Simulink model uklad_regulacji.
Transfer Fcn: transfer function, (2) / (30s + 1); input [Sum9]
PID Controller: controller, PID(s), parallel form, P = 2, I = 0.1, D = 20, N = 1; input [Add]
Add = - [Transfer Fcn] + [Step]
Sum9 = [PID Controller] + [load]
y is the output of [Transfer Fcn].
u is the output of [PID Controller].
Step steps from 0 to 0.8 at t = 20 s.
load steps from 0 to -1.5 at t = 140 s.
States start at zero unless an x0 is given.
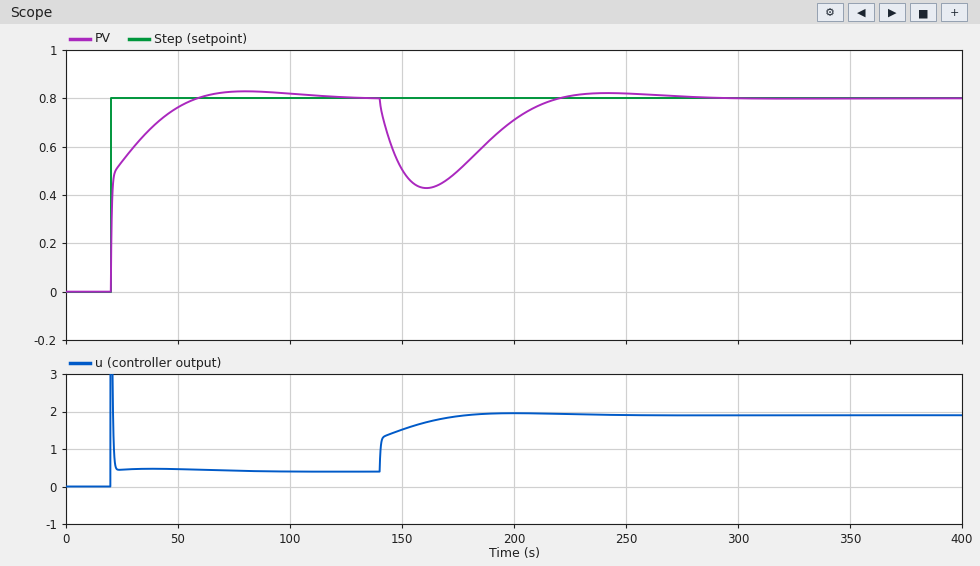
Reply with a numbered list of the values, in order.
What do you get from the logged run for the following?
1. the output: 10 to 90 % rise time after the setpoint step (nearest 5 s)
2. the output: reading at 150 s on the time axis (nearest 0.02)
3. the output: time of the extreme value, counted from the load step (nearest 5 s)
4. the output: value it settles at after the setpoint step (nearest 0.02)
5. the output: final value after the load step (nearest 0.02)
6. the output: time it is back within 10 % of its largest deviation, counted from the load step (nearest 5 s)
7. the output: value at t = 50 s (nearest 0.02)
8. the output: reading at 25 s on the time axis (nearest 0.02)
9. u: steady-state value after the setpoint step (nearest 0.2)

1. 25 s
2. 0.50
3. 20 s
4. 0.80
5. 0.80
6. 70 s
7. 0.76
8. 0.54
9. 0.4
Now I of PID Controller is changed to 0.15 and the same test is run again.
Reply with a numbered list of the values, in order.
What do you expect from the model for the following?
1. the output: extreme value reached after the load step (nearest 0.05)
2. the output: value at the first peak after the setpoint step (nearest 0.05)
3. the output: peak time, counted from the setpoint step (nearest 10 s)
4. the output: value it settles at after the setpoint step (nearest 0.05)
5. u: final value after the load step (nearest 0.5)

1. 0.45
2. 0.85
3. 50 s
4. 0.80
5. 2.0
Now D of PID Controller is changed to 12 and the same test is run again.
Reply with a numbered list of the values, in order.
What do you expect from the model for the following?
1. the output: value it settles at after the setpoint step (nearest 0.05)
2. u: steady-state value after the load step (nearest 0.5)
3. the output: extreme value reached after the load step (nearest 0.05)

1. 0.80
2. 2.0
3. 0.40
